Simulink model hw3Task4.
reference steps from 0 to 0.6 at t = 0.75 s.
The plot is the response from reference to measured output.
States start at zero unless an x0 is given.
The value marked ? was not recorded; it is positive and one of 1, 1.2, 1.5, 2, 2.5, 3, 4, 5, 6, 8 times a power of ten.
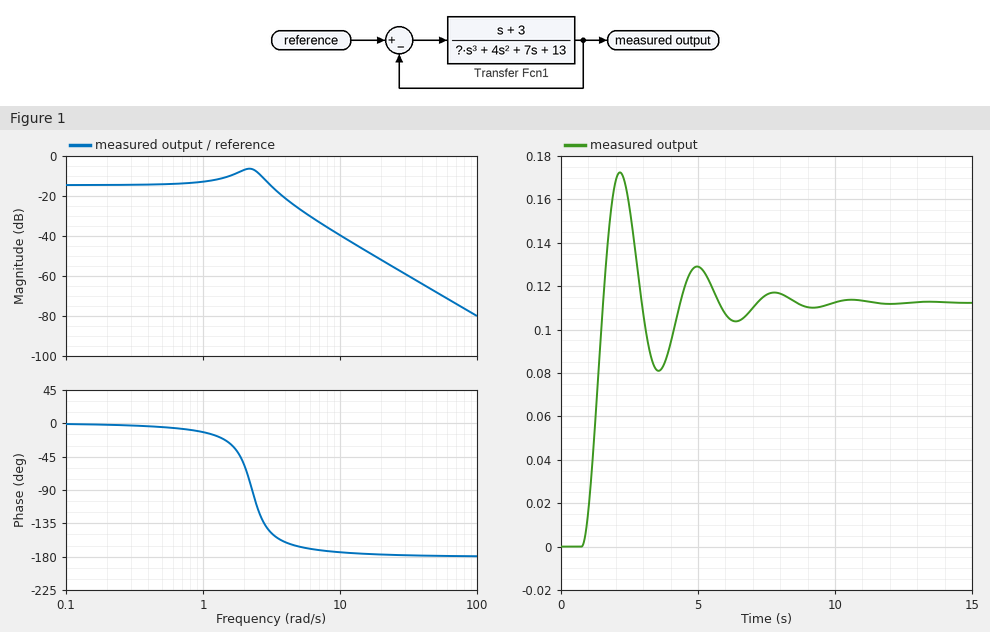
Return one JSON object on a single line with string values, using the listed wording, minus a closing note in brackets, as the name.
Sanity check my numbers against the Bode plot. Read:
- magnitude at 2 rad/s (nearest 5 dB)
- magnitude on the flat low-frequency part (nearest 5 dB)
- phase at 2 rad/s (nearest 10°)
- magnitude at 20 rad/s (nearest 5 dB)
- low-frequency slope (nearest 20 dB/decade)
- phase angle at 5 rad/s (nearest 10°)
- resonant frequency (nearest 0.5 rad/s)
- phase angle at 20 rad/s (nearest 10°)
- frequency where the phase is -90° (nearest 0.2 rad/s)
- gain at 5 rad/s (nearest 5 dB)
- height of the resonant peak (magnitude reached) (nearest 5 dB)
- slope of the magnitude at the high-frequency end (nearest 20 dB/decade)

{"magnitude at 2 rad/s": "-5 dB", "magnitude on the flat low-frequency part": "-15 dB", "phase at 2 rad/s": "-60°", "magnitude at 20 rad/s": "-50 dB", "low-frequency slope": "0 dB/decade", "phase angle at 5 rad/s": "-170°", "resonant frequency": "2.0 rad/s", "phase angle at 20 rad/s": "-180°", "frequency where the phase is -90°": "2.2 rad/s", "gain at 5 rad/s": "-25 dB", "height of the resonant peak (magnitude reached)": "-5 dB", "slope of the magnitude at the high-frequency end": "-40 dB/decade"}
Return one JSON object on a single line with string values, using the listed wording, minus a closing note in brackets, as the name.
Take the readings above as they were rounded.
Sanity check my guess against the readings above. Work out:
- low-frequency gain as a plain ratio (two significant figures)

{"low-frequency gain as a plain ratio": "0.18"}
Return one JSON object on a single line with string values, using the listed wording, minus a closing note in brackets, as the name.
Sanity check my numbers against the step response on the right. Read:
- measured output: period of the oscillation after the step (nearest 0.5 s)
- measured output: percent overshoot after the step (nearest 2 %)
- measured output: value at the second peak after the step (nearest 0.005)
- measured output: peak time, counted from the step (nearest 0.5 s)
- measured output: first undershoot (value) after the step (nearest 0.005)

{"measured output: period of the oscillation after the step": "3.0 s", "measured output: percent overshoot after the step": "54 %", "measured output: value at the second peak after the step": "0.130", "measured output: peak time, counted from the step": "1.5 s", "measured output: first undershoot (value) after the step": "0.080"}
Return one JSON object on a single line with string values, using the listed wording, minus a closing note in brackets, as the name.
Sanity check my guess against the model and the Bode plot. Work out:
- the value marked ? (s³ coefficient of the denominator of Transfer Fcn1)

{"the value marked ?": "1"}
